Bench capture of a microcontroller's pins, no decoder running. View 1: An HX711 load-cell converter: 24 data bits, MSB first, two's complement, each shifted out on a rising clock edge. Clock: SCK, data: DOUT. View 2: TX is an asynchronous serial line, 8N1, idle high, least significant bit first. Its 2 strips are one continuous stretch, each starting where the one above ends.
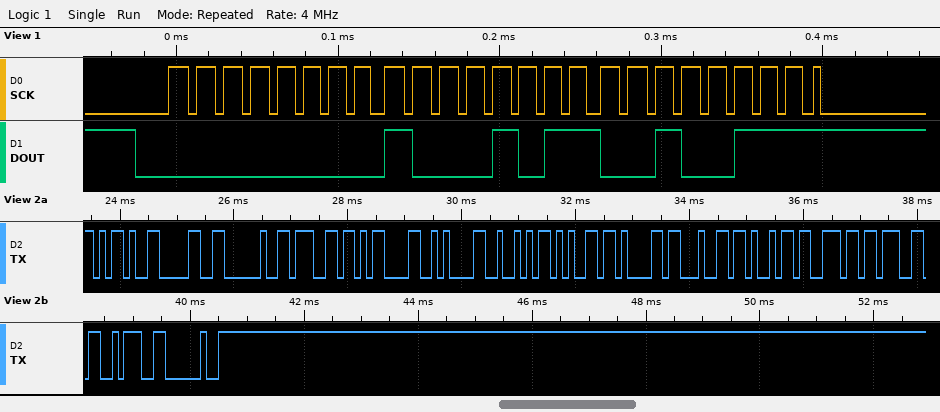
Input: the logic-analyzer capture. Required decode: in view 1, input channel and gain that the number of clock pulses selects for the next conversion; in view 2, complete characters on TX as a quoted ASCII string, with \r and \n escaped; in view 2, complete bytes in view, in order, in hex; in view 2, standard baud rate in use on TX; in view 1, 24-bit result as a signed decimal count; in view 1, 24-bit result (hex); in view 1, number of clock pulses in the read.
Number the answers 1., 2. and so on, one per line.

1. channel A, gain 128
2. "-0 g\r\nReading: "
3. 0x2D 0x30 0x20 0x67 0x0D 0x0A 0x52 0x65 0x61 0x64 0x69 0x6E 0x67 0x3A 0x20
4. 9600 baud
5. 35623
6. 0x008B27
7. 25
